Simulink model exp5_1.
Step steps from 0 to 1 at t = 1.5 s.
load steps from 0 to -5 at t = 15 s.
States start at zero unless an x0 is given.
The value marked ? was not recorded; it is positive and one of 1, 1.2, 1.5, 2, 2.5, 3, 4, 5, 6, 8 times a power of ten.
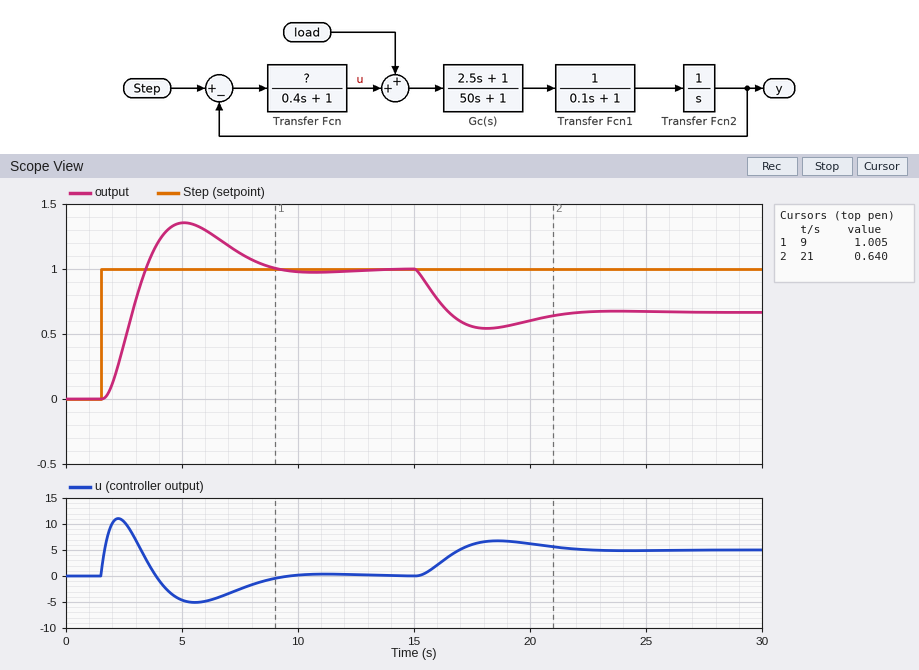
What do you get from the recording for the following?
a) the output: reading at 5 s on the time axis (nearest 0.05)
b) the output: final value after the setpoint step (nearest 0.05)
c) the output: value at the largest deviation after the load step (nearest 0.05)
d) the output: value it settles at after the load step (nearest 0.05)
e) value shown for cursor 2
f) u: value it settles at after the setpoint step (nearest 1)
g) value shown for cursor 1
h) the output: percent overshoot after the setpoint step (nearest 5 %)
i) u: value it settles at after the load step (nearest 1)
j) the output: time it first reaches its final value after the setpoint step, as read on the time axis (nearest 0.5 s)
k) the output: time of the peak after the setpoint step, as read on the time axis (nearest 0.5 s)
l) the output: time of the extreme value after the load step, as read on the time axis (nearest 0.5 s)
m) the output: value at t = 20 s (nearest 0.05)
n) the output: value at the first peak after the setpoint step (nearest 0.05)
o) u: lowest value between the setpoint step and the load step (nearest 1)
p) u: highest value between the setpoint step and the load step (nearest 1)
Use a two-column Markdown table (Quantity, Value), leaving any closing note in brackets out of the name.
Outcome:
| Quantity | Value |
|---|---|
| the output: reading at 5 s on the time axis | 1.35 |
| the output: final value after the setpoint step | 1.00 |
| the output: value at the largest deviation after the load step | 0.55 |
| the output: value it settles at after the load step | 0.65 |
| value shown for cursor 2 | 0.640 |
| u: value it settles at after the setpoint step | 0 |
| value shown for cursor 1 | 1.005 |
| the output: percent overshoot after the setpoint step | 35 % |
| u: value it settles at after the load step | 5 |
| the output: time it first reaches its final value after the setpoint step, as read on the time axis | 3.5 s |
| the output: time of the peak after the setpoint step, as read on the time axis | 5.0 s |
| the output: time of the extreme value after the load step, as read on the time axis | 18.0 s |
| the output: value at t = 20 s | 0.60 |
| the output: value at the first peak after the setpoint step | 1.35 |
| u: lowest value between the setpoint step and the load step | -5 |
| u: highest value between the setpoint step and the load step | 11 |
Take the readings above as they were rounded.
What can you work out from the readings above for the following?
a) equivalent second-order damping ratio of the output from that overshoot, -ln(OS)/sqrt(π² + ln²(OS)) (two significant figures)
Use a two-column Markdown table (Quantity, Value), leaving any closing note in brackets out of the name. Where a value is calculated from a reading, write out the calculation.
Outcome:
| Quantity | Value |
|---|---|
| equivalent second-order damping ratio of the output from that overshoot, -ln(OS)/sqrt(π² + ln²(OS)) | ln(0.35) = -1.050; 1.050 / sqrt(9.870 + 1.102) = 0.32 |
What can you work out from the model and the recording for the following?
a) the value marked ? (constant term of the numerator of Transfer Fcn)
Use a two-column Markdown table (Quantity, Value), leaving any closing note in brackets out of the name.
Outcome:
| Quantity | Value |
|---|---|
| the value marked ? | 15 |
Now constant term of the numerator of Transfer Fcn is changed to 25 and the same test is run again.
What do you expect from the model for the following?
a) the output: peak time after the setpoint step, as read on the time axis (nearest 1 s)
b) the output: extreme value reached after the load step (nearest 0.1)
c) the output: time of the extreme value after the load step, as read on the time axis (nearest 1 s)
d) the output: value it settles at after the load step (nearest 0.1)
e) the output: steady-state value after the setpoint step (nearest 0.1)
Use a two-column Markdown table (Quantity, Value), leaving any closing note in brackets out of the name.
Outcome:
| Quantity | Value |
|---|---|
| the output: peak time after the setpoint step, as read on the time axis | 4 s |
| the output: extreme value reached after the load step | 0.7 |
| the output: time of the extreme value after the load step, as read on the time axis | 17 s |
| the output: value it settles at after the load step | 0.8 |
| the output: steady-state value after the setpoint step | 1.0 |
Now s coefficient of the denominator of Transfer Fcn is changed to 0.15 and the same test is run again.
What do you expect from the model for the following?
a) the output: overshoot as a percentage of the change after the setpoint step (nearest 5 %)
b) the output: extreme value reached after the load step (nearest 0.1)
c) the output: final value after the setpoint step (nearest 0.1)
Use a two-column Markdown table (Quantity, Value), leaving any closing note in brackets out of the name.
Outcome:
| Quantity | Value |
|---|---|
| the output: overshoot as a percentage of the change after the setpoint step | 25 % |
| the output: extreme value reached after the load step | 0.6 |
| the output: final value after the setpoint step | 1.0 |
